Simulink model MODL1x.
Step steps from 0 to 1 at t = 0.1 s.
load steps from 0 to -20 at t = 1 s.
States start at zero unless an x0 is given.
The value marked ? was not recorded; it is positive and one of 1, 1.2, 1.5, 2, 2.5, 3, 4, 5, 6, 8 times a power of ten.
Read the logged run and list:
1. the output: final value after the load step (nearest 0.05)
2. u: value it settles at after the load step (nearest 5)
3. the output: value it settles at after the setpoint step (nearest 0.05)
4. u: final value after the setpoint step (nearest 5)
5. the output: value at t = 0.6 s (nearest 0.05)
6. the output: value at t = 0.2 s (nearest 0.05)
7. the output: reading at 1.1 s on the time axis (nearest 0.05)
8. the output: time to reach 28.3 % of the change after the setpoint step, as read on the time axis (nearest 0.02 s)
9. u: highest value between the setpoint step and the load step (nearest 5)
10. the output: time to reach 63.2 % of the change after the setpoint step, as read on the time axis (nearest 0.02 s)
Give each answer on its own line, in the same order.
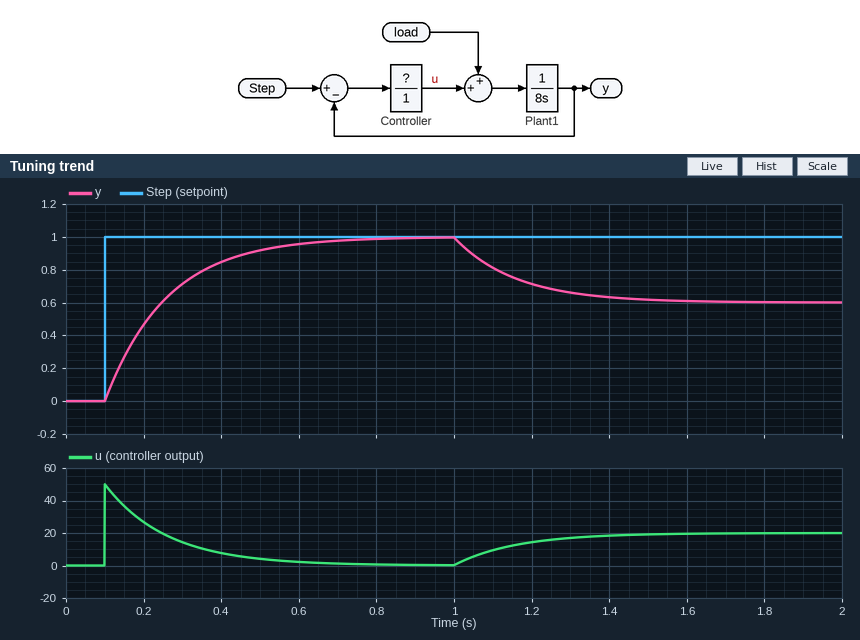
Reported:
0.60
20
1.00
0
0.95
0.45
0.80
0.16 s
50
0.26 s
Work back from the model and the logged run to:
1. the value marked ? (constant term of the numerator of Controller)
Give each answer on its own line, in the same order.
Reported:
50
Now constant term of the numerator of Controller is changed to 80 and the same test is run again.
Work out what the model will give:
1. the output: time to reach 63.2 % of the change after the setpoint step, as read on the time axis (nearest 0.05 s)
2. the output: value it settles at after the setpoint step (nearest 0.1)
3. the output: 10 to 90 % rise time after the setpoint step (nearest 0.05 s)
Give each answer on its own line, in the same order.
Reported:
0.20 s
1.0
0.20 s
